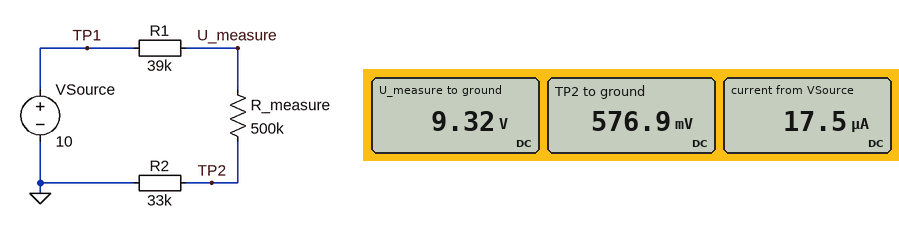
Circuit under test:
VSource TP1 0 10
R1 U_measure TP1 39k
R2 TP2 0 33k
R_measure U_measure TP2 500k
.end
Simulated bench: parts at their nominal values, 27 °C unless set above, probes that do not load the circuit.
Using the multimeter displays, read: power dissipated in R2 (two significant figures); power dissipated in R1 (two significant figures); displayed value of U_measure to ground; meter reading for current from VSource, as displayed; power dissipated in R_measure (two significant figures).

10 µW
12 µW
9.32 V
17.5 µA
150 µW
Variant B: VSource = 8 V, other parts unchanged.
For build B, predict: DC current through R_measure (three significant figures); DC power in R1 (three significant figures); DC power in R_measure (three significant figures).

14.0 µA
7.63 µW
97.8 µW
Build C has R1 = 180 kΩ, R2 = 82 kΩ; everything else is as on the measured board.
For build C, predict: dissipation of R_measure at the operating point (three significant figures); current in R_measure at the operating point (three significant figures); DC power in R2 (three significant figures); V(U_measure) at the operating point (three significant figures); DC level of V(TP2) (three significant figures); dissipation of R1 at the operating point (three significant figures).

86.1 µW
13.1 µA
14.1 µW
7.64 V
1.08 V
31.0 µW
